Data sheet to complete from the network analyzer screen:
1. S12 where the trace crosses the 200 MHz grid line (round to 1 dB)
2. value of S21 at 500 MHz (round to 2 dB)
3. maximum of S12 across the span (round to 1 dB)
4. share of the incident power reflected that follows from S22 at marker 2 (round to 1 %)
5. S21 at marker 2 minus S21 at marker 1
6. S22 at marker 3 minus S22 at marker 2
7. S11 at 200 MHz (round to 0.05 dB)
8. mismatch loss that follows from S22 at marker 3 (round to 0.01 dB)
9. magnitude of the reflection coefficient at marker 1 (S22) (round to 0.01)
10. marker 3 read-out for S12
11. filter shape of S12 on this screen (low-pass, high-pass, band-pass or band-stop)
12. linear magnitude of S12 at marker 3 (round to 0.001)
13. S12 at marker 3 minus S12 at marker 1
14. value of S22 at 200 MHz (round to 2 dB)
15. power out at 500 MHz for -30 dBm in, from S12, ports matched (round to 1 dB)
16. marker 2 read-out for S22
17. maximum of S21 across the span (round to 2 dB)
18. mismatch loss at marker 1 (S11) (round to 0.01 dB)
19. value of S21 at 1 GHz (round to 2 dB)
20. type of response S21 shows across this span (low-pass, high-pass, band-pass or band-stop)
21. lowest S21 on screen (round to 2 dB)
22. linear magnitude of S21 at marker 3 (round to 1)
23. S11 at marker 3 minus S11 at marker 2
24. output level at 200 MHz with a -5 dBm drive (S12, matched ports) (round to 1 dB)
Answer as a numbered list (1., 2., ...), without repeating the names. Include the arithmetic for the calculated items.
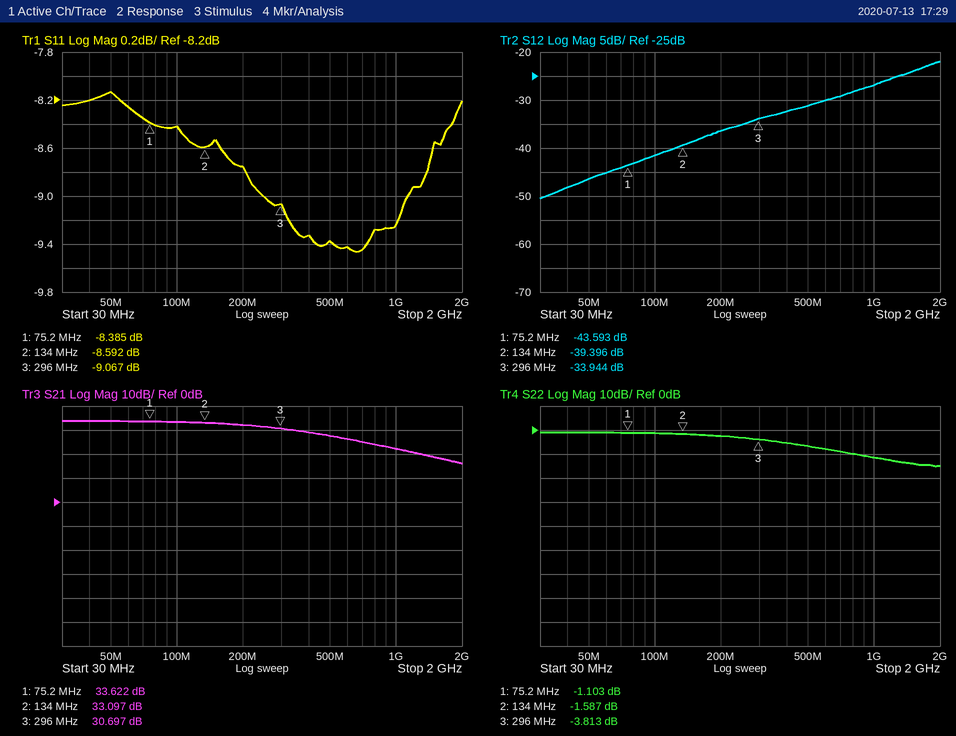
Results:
1. -36 dB
2. 28 dB
3. -22 dB
4. 10^(-1.587/10) ≈ 69 %
5. 33.097 − (33.622) = -0.525 dB
6. -3.813 − (-1.587) = -2.226 dB
7. -8.75 dB
8. −10 log10(1 − 10^(-3.813/10)) ≈ 2.33 dB
9. 10^(-1.103/20) ≈ 0.88
10. -33.944 dB
11. high-pass
12. 10^(-33.944/20) ≈ 0.020
13. -33.944 − (-43.593) = 9.649 dB
14. -2 dB
15. -30 dBm + (-31 dB) = -61 dBm
16. -1.587 dB
17. 34 dB
18. −10 log10(1 − 10^(-8.385/10)) ≈ 0.68 dB
19. 22 dB
20. low-pass
21. 16 dB
22. 10^(30.697/20) ≈ 34
23. -9.067 − (-8.592) = -0.475 dB
24. -5 dBm + (-36 dB) = -41 dBm
